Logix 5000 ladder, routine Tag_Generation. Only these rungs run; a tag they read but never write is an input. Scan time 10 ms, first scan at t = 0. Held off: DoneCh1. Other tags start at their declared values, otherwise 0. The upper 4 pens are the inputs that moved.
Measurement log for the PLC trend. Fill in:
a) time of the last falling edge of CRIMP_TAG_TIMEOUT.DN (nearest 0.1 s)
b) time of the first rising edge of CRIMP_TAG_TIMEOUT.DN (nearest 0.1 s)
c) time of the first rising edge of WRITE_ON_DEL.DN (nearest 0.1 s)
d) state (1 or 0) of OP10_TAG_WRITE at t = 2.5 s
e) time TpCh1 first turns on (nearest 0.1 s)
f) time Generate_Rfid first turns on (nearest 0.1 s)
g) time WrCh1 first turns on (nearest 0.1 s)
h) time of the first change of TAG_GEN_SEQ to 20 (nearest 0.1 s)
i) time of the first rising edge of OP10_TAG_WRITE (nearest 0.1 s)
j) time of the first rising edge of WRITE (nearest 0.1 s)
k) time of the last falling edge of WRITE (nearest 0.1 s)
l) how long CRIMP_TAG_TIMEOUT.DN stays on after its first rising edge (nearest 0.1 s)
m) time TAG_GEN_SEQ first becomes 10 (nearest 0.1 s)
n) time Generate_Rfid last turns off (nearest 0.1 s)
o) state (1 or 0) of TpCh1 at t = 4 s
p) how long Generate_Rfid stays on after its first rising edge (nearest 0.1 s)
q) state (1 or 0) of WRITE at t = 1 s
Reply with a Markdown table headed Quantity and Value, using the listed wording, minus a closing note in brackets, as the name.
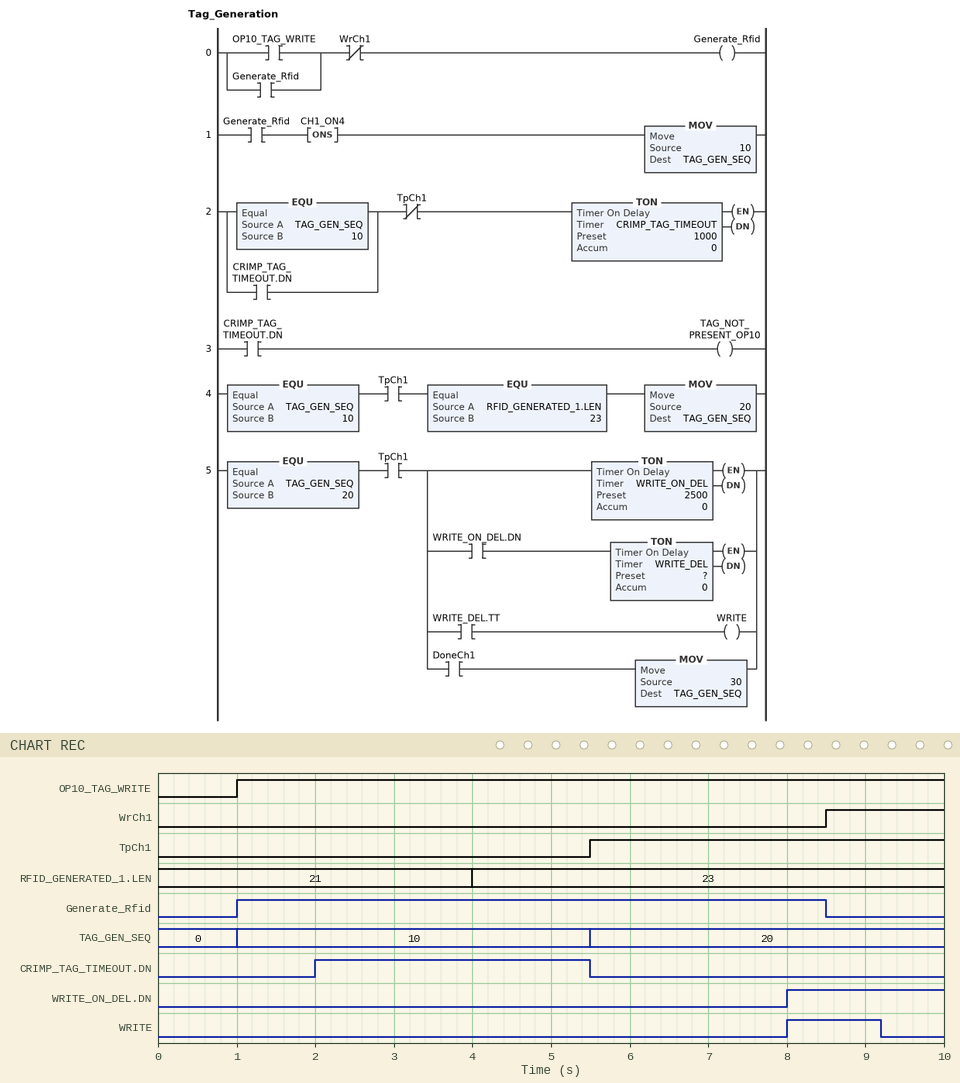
| Quantity | Value |
|---|---|
| time of the last falling edge of CRIMP_TAG_TIMEOUT.DN | 5.5 s |
| time of the first rising edge of CRIMP_TAG_TIMEOUT.DN | 2.0 s |
| time of the first rising edge of WRITE_ON_DEL.DN | 8.0 s |
| state (1 or 0) of OP10_TAG_WRITE at t = 2.5 s | 1 |
| time TpCh1 first turns on | 5.5 s |
| time Generate_Rfid first turns on | 1.0 s |
| time WrCh1 first turns on | 8.5 s |
| time of the first change of TAG_GEN_SEQ to 20 | 5.5 s |
| time of the first rising edge of OP10_TAG_WRITE | 1.0 s |
| time of the first rising edge of WRITE | 8.0 s |
| time of the last falling edge of WRITE | 9.2 s |
| how long CRIMP_TAG_TIMEOUT.DN stays on after its first rising edge | 3.5 s |
| time TAG_GEN_SEQ first becomes 10 | 1.0 s |
| time Generate_Rfid last turns off | 8.5 s |
| state (1 or 0) of TpCh1 at t = 4 s | 0 |
| how long Generate_Rfid stays on after its first rising edge | 7.5 s |
| state (1 or 0) of WRITE at t = 1 s | 0 |
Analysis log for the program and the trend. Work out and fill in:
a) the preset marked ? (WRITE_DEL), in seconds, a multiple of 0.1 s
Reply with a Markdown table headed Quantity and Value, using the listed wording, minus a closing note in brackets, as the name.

| Quantity | Value |
|---|---|
| the preset marked ? (WRITE_DEL), in seconds, a multiple of 0.1 s | 1.2 s |
